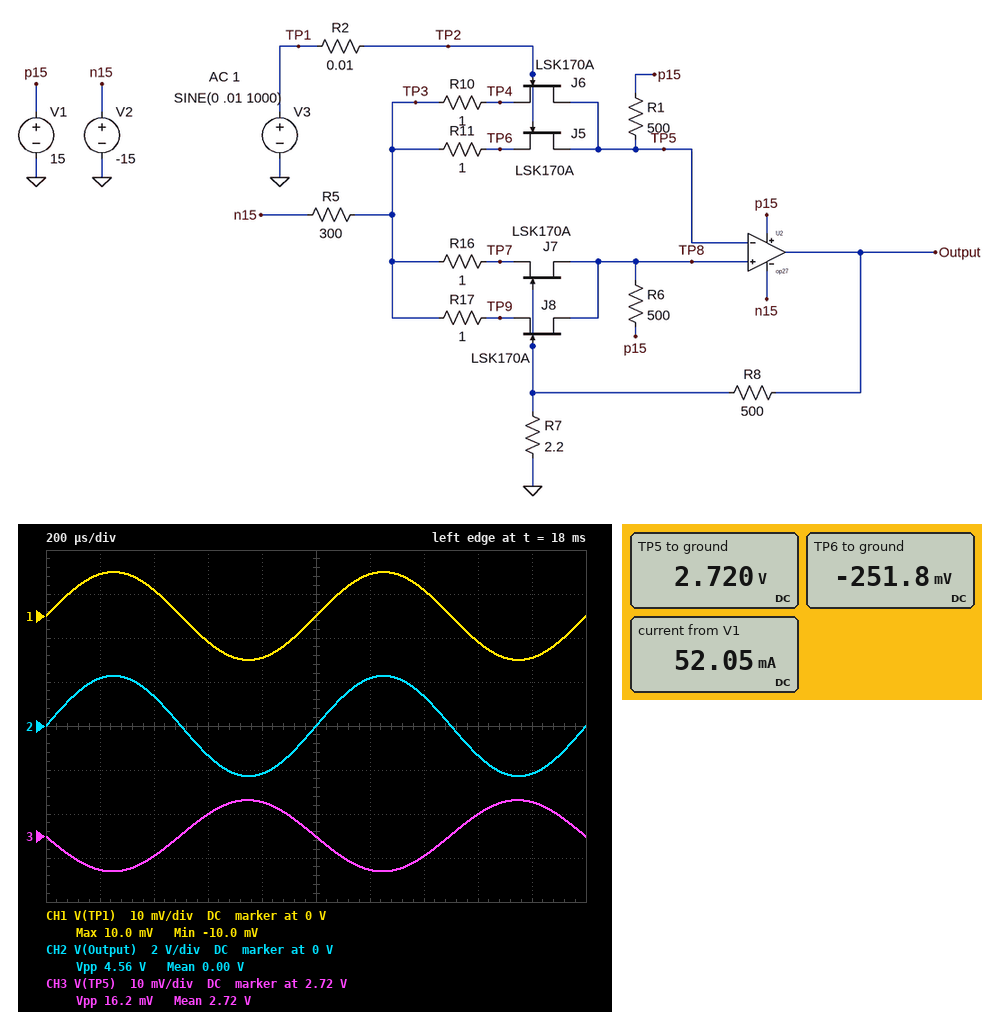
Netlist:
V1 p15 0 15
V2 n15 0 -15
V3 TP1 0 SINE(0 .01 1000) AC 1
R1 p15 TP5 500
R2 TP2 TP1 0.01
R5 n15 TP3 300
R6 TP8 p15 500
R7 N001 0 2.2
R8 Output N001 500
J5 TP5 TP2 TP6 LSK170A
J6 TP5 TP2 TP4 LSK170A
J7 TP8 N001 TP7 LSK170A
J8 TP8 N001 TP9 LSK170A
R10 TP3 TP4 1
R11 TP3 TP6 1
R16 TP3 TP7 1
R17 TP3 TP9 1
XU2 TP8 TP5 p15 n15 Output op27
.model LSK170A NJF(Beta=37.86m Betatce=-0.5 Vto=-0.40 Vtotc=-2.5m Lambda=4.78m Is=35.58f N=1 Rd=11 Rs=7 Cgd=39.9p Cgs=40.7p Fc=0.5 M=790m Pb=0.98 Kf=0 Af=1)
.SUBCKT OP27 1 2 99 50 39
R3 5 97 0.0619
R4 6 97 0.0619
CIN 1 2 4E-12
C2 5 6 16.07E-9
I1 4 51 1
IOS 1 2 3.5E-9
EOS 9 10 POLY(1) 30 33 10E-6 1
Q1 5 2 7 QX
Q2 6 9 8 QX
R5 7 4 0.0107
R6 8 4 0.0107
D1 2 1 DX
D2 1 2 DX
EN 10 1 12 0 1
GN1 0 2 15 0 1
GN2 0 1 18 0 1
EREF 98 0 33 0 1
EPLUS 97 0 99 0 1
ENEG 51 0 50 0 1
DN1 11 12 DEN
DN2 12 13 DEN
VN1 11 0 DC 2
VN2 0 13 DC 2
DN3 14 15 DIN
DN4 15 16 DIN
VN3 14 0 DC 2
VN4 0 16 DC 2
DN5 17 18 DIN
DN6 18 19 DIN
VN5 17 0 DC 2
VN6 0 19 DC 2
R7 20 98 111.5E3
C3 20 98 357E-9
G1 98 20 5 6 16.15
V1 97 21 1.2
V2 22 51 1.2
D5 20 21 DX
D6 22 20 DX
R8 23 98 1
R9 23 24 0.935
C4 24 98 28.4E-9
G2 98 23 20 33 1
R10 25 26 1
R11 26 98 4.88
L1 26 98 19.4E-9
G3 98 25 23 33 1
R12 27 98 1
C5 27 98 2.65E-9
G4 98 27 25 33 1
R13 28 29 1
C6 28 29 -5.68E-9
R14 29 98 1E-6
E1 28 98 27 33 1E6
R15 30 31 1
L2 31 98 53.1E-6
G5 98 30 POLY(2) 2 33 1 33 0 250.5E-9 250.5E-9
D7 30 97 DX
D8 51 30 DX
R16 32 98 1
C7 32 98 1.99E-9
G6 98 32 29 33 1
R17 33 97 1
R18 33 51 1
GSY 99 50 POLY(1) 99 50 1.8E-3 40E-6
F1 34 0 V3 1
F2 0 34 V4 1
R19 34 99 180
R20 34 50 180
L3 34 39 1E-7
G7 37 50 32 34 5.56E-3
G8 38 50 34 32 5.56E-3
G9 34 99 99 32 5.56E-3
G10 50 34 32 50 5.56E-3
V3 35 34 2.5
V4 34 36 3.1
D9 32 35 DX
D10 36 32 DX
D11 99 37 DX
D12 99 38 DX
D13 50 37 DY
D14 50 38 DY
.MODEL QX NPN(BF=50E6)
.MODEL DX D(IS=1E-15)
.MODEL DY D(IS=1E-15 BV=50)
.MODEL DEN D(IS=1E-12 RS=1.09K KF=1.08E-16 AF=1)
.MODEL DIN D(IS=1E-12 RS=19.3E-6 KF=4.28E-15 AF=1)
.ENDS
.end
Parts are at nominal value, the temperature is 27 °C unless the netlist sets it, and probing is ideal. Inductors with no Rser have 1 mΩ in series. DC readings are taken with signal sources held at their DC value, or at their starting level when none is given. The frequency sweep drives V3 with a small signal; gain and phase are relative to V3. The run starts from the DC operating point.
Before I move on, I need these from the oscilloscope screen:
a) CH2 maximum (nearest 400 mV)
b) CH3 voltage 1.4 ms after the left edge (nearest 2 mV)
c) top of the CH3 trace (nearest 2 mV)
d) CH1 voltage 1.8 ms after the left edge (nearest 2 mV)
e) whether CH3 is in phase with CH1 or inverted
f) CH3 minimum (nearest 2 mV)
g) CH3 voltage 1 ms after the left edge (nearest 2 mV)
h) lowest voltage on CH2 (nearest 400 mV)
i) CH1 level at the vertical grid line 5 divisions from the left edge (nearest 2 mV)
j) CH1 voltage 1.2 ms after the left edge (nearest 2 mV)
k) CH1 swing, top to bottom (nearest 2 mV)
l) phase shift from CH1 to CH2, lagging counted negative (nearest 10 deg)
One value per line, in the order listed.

2.4 V
2.716 V
2.728 V
-10 mV
inverted
2.712 V
2.720 V
-2.4 V
0 V
10 mV
20 mV
0 deg
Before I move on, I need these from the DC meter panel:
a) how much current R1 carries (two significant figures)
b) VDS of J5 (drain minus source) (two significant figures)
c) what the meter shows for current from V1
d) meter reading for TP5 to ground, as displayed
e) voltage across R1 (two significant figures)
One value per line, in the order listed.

25 mA
3.0 V
52.05 mA
2.720 V
12 V
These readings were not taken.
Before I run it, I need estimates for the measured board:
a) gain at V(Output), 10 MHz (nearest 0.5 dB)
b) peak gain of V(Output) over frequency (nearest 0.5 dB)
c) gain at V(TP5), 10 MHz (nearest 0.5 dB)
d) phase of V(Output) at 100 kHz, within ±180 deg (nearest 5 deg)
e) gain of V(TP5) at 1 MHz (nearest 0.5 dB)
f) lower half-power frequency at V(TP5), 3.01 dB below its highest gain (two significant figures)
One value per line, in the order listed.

20.0 dB
47.0 dB
19.0 dB
-5 deg
23.0 dB
750 kHz
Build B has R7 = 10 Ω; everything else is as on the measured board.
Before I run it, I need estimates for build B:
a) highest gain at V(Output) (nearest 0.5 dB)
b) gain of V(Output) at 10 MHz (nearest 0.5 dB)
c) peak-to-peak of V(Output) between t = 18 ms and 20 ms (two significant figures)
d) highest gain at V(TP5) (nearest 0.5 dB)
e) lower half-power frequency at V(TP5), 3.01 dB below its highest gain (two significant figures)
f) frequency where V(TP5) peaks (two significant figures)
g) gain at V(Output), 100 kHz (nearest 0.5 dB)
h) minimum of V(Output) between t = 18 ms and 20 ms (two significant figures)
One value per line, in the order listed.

36.0 dB
20.0 dB
1.0 V
26.0 dB
2.4 MHz
3.7 MHz
34.0 dB
-510 mV
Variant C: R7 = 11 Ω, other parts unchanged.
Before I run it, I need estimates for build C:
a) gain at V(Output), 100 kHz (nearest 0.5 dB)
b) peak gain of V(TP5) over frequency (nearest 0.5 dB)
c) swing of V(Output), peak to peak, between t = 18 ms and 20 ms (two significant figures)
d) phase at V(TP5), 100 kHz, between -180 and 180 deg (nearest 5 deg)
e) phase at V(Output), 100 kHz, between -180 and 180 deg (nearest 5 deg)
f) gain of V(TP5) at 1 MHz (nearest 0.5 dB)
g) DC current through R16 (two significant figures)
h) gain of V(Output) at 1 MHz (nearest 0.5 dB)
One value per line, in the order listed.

33.5 dB
26.0 dB
930 mV
-155 deg
0 deg
12.0 dB
12 mA
34.0 dB
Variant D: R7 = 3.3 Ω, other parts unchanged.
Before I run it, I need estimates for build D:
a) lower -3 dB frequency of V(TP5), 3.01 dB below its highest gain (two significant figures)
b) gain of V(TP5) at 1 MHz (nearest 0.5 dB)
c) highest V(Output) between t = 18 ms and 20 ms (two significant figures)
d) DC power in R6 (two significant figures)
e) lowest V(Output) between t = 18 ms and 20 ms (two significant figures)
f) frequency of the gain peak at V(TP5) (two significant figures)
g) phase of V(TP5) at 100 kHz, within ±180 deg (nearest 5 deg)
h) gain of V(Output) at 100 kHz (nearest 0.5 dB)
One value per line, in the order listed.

1.1 MHz
21.5 dB
1.5 V
300 mW
-1.5 V
2.3 MHz
-125 deg
43.5 dB
